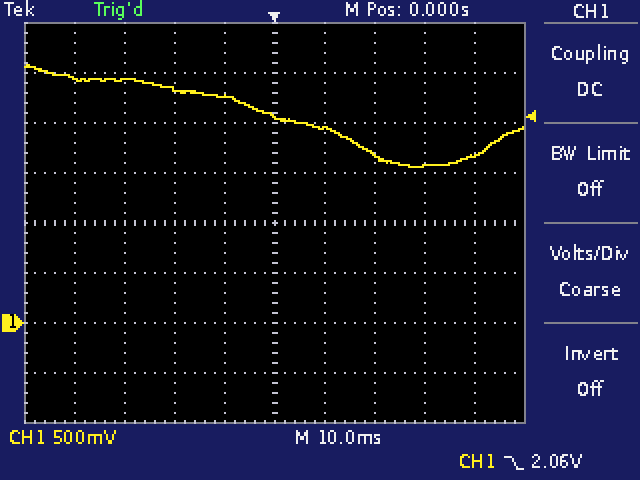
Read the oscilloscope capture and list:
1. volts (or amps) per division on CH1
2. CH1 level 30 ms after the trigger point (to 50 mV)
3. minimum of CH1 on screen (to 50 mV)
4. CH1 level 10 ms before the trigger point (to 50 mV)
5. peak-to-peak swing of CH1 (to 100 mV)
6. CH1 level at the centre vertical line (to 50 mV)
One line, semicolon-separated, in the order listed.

500 mV; 1.55 V; 1.55 V; 2.25 V; 1.00 V; 2.05 V
